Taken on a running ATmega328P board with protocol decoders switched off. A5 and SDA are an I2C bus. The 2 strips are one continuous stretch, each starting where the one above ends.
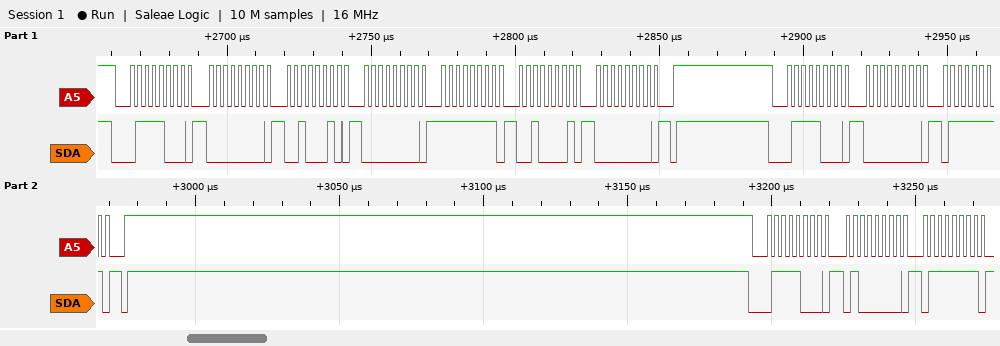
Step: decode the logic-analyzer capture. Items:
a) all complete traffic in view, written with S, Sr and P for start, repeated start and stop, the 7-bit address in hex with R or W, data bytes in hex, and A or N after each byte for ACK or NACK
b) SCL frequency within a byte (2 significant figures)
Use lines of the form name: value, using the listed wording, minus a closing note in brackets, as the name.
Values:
all complete traffic in view, written with S, Sr and P for start, repeated start and stop, the 7-bit address in hex with R or W, data bytes in hex, and A or N after each byte for ACK or NACK: S 3CW A 00 A 22 A 00 A FF A 21 A 00 A P S 3CW A 00 A 7F A P S 3CW A 40 A 7F A
SCL frequency within a byte: 400 kHz
